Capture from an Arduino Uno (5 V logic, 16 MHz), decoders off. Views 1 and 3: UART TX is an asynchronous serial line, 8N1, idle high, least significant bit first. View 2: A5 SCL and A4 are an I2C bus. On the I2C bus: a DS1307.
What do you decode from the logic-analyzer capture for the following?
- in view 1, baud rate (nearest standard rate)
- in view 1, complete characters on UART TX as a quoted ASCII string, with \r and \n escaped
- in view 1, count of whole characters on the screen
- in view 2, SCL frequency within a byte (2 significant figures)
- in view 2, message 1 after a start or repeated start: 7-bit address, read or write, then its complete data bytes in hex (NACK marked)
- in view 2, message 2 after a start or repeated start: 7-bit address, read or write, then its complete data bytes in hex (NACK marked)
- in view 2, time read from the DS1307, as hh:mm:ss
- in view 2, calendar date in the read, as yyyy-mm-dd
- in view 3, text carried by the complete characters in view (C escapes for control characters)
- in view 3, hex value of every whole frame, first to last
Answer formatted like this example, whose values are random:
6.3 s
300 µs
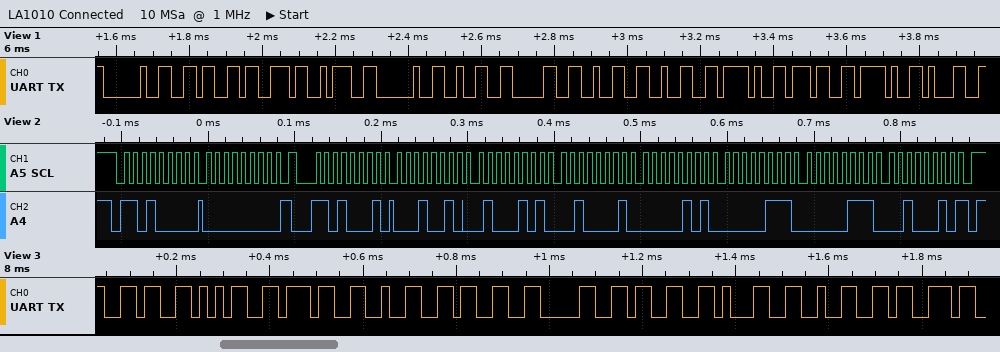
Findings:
57600 baud
" 6s: 2022/7/1"
13
100 kHz
0x68 write: 00
0x68 read: 12 45 21 05 07 07 22 NACK
21:45:12
2022-07-07
"657230312s"
0x36 0x35 0x37 0x32 0x33 0x30 0x33 0x31 0x32 0x73
